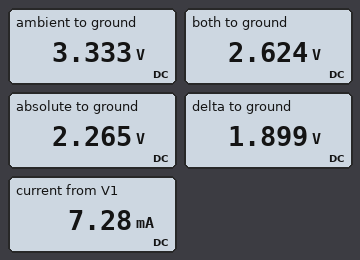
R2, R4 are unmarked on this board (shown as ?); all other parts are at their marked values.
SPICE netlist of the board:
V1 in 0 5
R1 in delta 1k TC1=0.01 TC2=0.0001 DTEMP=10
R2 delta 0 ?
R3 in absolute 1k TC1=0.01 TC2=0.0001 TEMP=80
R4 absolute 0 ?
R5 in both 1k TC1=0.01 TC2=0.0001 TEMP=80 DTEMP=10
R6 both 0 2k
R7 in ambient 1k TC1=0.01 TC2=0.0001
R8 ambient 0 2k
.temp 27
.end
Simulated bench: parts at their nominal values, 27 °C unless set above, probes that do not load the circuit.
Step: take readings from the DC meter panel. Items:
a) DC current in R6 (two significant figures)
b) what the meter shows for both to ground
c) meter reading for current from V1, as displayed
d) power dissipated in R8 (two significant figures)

1.3 mA
2.624 V
7.28 mA
5.6 mW
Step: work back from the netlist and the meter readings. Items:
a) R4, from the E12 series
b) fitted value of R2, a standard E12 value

1.5 kΩ
680 Ω
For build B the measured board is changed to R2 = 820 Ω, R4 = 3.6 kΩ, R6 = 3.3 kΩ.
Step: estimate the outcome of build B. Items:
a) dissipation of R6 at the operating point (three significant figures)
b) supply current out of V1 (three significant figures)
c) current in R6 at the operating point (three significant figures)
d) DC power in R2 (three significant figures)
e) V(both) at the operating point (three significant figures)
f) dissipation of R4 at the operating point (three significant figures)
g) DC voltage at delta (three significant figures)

3.16 mW
6.16 mA
978 µA
5.50 mW
3.23 V
3.07 mW
2.12 V
